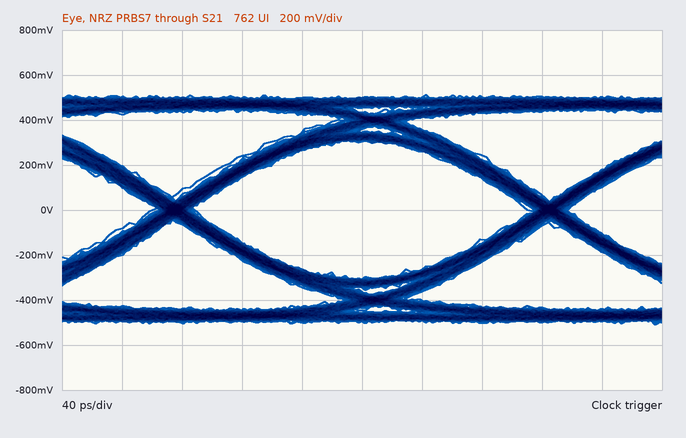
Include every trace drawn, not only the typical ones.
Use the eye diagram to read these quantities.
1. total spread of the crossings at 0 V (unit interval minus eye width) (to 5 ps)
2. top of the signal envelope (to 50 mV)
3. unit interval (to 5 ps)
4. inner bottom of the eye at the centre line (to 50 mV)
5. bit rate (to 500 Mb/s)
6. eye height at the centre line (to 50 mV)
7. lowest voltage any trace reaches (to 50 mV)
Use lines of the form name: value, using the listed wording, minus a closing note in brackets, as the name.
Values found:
total spread of the crossings at 0 V (unit interval minus eye width): 30 ps
top of the signal envelope: 500 mV
unit interval: 250 ps
inner bottom of the eye at the centre line: -300 mV
bit rate: 4.0 Gb/s
eye height at the centre line: 600 mV
lowest voltage any trace reaches: -500 mV
